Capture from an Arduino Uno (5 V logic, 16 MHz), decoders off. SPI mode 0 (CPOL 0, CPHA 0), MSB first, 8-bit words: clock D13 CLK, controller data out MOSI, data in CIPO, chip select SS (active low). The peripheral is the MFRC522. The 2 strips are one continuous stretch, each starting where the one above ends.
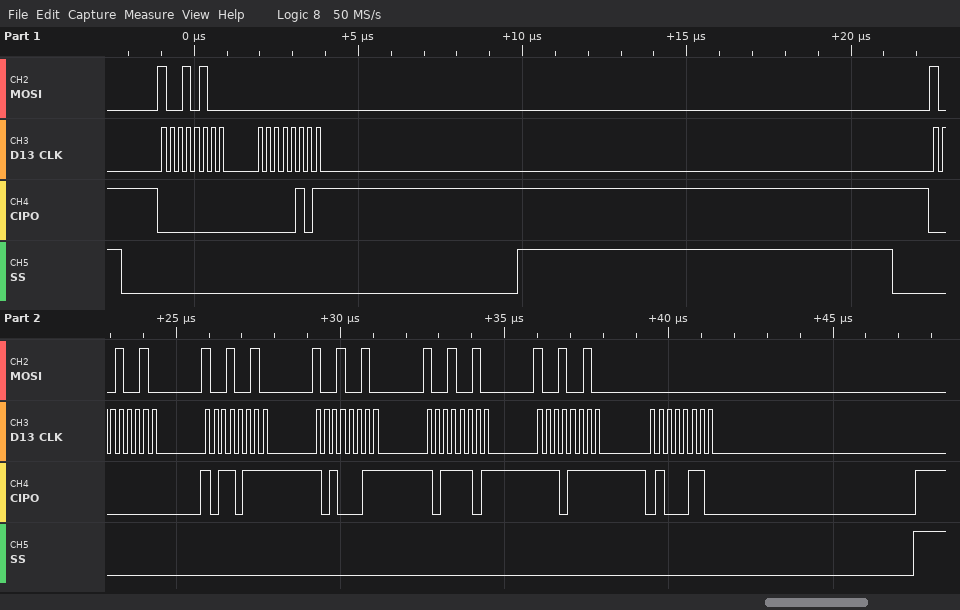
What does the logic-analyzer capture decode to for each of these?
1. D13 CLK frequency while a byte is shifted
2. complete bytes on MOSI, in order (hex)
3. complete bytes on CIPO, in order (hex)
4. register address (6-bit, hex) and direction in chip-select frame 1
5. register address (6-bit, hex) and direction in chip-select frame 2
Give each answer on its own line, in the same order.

4 MHz
94 00 92 92 92 92 92 00
00 05 00 B7 A3 BD EF 46
0x0A read
0x09 read
